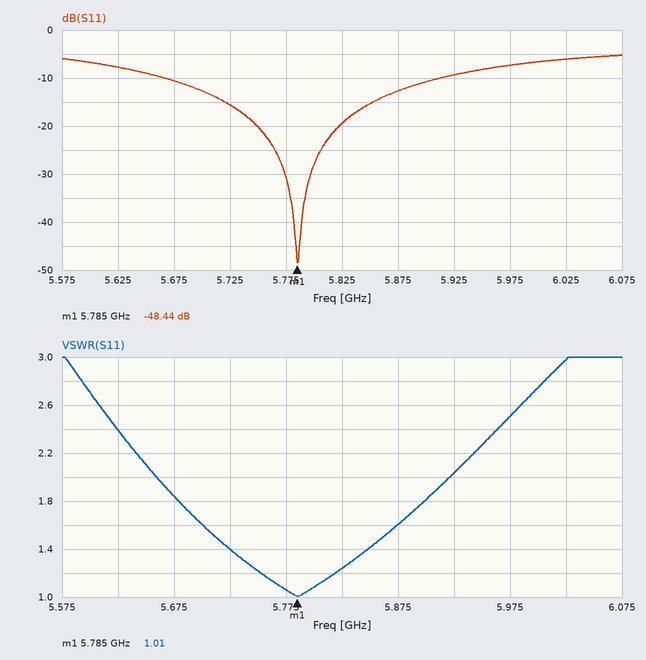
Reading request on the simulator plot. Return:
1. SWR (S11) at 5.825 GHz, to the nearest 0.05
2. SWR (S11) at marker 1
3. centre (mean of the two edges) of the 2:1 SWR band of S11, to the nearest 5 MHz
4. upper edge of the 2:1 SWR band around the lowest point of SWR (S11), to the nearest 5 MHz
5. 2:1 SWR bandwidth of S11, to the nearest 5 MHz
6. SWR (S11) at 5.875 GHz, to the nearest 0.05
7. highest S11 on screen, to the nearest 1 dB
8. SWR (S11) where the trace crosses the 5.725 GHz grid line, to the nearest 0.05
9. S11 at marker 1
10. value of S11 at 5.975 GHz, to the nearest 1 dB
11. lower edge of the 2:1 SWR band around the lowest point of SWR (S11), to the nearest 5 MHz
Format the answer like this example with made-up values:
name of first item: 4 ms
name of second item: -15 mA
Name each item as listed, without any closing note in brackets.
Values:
SWR (S11) at 5.825 GHz, to the nearest 0.05: 1.25
SWR (S11) at marker 1: 1.01
centre (mean of the two edges) of the 2:1 SWR band of S11, to the nearest 5 MHz: 5.790 GHz
upper edge of the 2:1 SWR band around the lowest point of SWR (S11), to the nearest 5 MHz: 5.920 GHz
2:1 SWR bandwidth of S11, to the nearest 5 MHz: 260 MHz
SWR (S11) at 5.875 GHz, to the nearest 0.05: 1.60
highest S11 on screen, to the nearest 1 dB: -5 dB
SWR (S11) where the trace crosses the 5.725 GHz grid line, to the nearest 0.05: 1.40
S11 at marker 1: -48.44 dB
value of S11 at 5.975 GHz, to the nearest 1 dB: -7 dB
lower edge of the 2:1 SWR band around the lowest point of SWR (S11), to the nearest 5 MHz: 5.660 GHz
